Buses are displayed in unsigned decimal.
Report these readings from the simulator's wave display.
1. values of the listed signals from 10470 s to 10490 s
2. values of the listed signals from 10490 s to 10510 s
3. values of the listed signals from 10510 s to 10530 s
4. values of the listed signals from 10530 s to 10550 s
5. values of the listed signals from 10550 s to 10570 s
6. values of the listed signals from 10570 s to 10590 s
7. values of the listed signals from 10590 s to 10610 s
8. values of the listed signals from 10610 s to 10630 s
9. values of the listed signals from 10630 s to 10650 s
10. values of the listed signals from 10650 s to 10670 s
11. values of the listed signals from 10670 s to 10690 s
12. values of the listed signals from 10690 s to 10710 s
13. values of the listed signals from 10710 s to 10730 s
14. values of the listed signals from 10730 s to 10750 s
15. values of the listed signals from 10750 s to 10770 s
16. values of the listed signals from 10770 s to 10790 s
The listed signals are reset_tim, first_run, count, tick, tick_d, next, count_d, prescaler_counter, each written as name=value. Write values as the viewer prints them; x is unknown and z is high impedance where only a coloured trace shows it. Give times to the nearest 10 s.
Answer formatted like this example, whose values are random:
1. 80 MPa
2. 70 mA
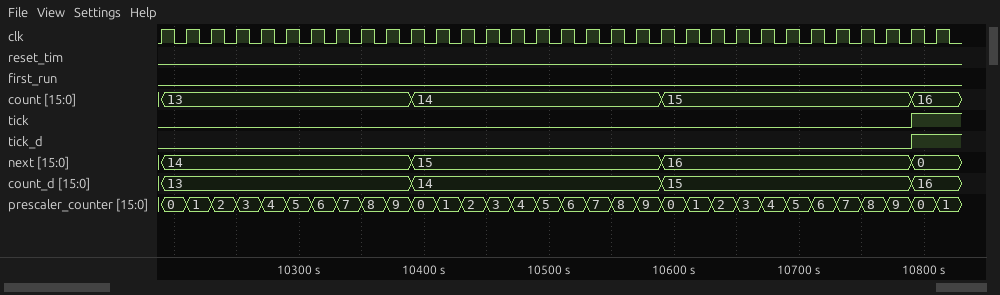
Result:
1. reset_tim=0, first_run=0, count=14, tick=0, tick_d=0, next=15, count_d=14, prescaler_counter=4
2. reset_tim=0, first_run=0, count=14, tick=0, tick_d=0, next=15, count_d=14, prescaler_counter=5
3. reset_tim=0, first_run=0, count=14, tick=0, tick_d=0, next=15, count_d=14, prescaler_counter=6
4. reset_tim=0, first_run=0, count=14, tick=0, tick_d=0, next=15, count_d=14, prescaler_counter=7
5. reset_tim=0, first_run=0, count=14, tick=0, tick_d=0, next=15, count_d=14, prescaler_counter=8
6. reset_tim=0, first_run=0, count=14, tick=0, tick_d=0, next=15, count_d=14, prescaler_counter=9
7. reset_tim=0, first_run=0, count=15, tick=0, tick_d=0, next=16, count_d=15, prescaler_counter=0
8. reset_tim=0, first_run=0, count=15, tick=0, tick_d=0, next=16, count_d=15, prescaler_counter=1
9. reset_tim=0, first_run=0, count=15, tick=0, tick_d=0, next=16, count_d=15, prescaler_counter=2
10. reset_tim=0, first_run=0, count=15, tick=0, tick_d=0, next=16, count_d=15, prescaler_counter=3
11. reset_tim=0, first_run=0, count=15, tick=0, tick_d=0, next=16, count_d=15, prescaler_counter=4
12. reset_tim=0, first_run=0, count=15, tick=0, tick_d=0, next=16, count_d=15, prescaler_counter=5
13. reset_tim=0, first_run=0, count=15, tick=0, tick_d=0, next=16, count_d=15, prescaler_counter=6
14. reset_tim=0, first_run=0, count=15, tick=0, tick_d=0, next=16, count_d=15, prescaler_counter=7
15. reset_tim=0, first_run=0, count=15, tick=0, tick_d=0, next=16, count_d=15, prescaler_counter=8
16. reset_tim=0, first_run=0, count=15, tick=0, tick_d=0, next=16, count_d=15, prescaler_counter=9
